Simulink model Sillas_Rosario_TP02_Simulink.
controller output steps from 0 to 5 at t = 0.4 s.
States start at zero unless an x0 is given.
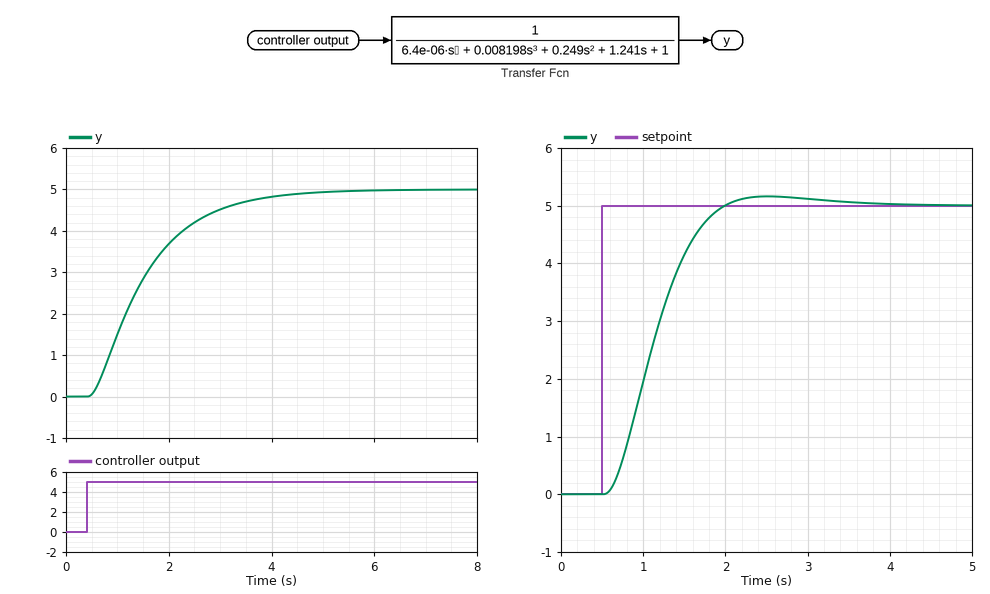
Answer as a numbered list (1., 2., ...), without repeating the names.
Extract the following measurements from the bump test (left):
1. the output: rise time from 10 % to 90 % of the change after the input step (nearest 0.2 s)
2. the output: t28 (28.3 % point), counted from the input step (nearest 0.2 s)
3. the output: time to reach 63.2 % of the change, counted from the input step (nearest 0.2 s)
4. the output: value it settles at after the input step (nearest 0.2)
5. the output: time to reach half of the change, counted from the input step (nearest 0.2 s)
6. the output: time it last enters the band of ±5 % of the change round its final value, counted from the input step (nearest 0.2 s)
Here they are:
1. 2.2 s
2. 0.6 s
3. 1.2 s
4. 5.0
5. 1.0 s
6. 3.2 s
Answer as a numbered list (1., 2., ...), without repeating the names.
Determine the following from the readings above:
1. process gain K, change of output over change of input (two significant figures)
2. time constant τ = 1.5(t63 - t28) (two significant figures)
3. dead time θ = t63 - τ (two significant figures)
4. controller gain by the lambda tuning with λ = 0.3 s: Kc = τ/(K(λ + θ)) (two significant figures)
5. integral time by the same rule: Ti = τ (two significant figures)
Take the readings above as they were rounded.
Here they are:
1. 1.0
2. 0.90 s
3. 0.30 s
4. 1.5
5. 0.90 s
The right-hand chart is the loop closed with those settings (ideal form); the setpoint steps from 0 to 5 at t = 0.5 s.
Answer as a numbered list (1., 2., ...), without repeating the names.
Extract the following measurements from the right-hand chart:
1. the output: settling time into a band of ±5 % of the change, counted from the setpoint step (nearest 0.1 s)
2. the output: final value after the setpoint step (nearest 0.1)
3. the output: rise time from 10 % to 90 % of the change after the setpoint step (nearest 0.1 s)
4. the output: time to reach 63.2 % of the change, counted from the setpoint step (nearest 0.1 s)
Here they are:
1. 1.3 s
2. 5.0
3. 0.9 s
4. 0.7 s
